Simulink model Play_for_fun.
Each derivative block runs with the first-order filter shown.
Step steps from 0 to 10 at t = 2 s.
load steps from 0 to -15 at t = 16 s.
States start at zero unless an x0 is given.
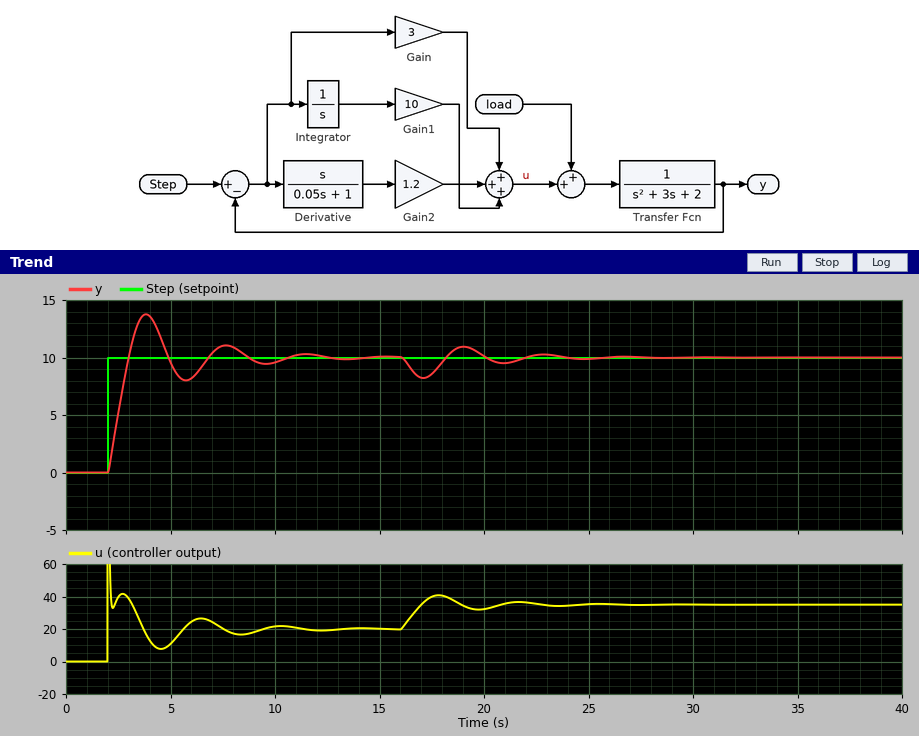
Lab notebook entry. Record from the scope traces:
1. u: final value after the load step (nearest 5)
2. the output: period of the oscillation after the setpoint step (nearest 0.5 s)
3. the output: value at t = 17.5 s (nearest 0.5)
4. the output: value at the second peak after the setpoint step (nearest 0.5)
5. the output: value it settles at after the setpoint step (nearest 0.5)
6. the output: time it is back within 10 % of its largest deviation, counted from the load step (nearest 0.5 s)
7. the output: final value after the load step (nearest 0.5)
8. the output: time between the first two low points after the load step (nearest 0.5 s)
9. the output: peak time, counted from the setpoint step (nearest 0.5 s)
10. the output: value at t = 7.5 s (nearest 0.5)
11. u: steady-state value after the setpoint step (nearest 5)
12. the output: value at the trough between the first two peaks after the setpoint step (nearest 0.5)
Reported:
35
4.0 s
8.5
11.0
10.0
7.5 s
10.0
4.0 s
2.0 s
11.0
20
8.0
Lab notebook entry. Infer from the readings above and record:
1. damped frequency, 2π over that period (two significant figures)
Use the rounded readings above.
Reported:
1.6 rad/s
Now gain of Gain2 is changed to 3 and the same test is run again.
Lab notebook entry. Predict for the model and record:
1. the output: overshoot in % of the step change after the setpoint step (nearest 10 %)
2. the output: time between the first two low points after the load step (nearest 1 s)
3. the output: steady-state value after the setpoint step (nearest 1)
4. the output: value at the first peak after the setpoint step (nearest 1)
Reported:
20 %
5 s
10
12
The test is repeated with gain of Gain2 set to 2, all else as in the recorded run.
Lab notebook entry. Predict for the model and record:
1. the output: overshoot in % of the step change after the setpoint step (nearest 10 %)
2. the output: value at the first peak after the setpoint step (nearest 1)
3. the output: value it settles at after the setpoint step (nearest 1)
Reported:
30 %
13
10
